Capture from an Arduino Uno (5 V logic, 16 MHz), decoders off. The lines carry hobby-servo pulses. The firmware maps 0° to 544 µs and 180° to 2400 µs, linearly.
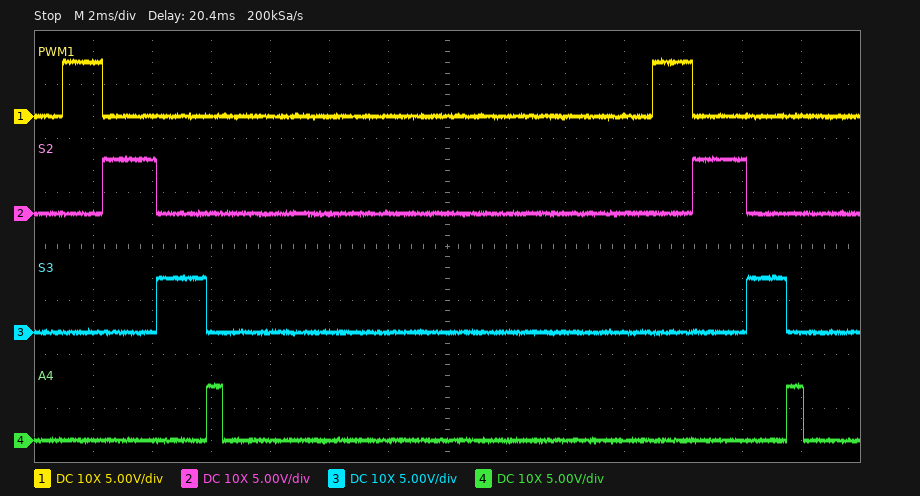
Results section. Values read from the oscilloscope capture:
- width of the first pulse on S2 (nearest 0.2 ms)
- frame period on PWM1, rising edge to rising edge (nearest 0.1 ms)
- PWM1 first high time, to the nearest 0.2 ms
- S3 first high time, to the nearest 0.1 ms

1.8 ms
20.0 ms
1.4 ms
1.7 ms
